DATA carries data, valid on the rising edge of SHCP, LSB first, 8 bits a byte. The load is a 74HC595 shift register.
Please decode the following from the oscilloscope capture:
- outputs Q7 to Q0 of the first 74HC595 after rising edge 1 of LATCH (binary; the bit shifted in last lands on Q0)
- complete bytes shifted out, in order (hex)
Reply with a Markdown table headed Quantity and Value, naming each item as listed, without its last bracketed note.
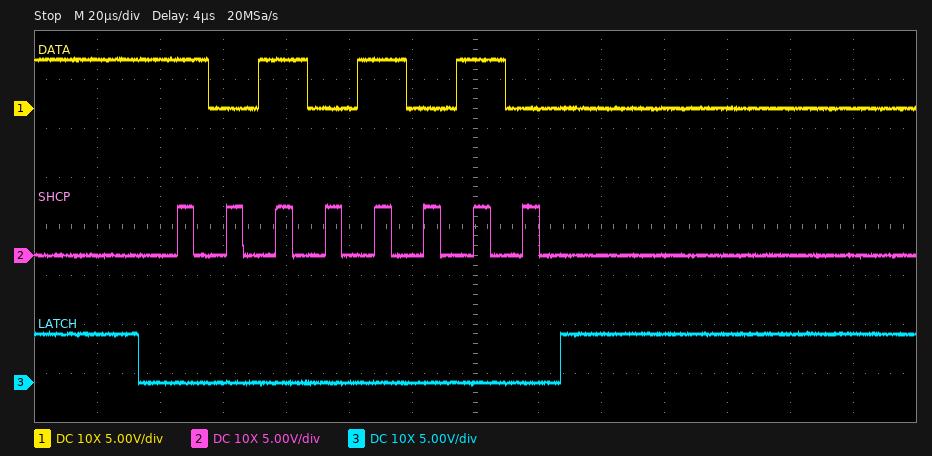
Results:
| Quantity | Value |
|---|---|
| outputs Q7 to Q0 of the first 74HC595 after rising edge 1 of LATCH | 10101010 |
| complete bytes shifted out, in order | 0x55 |
